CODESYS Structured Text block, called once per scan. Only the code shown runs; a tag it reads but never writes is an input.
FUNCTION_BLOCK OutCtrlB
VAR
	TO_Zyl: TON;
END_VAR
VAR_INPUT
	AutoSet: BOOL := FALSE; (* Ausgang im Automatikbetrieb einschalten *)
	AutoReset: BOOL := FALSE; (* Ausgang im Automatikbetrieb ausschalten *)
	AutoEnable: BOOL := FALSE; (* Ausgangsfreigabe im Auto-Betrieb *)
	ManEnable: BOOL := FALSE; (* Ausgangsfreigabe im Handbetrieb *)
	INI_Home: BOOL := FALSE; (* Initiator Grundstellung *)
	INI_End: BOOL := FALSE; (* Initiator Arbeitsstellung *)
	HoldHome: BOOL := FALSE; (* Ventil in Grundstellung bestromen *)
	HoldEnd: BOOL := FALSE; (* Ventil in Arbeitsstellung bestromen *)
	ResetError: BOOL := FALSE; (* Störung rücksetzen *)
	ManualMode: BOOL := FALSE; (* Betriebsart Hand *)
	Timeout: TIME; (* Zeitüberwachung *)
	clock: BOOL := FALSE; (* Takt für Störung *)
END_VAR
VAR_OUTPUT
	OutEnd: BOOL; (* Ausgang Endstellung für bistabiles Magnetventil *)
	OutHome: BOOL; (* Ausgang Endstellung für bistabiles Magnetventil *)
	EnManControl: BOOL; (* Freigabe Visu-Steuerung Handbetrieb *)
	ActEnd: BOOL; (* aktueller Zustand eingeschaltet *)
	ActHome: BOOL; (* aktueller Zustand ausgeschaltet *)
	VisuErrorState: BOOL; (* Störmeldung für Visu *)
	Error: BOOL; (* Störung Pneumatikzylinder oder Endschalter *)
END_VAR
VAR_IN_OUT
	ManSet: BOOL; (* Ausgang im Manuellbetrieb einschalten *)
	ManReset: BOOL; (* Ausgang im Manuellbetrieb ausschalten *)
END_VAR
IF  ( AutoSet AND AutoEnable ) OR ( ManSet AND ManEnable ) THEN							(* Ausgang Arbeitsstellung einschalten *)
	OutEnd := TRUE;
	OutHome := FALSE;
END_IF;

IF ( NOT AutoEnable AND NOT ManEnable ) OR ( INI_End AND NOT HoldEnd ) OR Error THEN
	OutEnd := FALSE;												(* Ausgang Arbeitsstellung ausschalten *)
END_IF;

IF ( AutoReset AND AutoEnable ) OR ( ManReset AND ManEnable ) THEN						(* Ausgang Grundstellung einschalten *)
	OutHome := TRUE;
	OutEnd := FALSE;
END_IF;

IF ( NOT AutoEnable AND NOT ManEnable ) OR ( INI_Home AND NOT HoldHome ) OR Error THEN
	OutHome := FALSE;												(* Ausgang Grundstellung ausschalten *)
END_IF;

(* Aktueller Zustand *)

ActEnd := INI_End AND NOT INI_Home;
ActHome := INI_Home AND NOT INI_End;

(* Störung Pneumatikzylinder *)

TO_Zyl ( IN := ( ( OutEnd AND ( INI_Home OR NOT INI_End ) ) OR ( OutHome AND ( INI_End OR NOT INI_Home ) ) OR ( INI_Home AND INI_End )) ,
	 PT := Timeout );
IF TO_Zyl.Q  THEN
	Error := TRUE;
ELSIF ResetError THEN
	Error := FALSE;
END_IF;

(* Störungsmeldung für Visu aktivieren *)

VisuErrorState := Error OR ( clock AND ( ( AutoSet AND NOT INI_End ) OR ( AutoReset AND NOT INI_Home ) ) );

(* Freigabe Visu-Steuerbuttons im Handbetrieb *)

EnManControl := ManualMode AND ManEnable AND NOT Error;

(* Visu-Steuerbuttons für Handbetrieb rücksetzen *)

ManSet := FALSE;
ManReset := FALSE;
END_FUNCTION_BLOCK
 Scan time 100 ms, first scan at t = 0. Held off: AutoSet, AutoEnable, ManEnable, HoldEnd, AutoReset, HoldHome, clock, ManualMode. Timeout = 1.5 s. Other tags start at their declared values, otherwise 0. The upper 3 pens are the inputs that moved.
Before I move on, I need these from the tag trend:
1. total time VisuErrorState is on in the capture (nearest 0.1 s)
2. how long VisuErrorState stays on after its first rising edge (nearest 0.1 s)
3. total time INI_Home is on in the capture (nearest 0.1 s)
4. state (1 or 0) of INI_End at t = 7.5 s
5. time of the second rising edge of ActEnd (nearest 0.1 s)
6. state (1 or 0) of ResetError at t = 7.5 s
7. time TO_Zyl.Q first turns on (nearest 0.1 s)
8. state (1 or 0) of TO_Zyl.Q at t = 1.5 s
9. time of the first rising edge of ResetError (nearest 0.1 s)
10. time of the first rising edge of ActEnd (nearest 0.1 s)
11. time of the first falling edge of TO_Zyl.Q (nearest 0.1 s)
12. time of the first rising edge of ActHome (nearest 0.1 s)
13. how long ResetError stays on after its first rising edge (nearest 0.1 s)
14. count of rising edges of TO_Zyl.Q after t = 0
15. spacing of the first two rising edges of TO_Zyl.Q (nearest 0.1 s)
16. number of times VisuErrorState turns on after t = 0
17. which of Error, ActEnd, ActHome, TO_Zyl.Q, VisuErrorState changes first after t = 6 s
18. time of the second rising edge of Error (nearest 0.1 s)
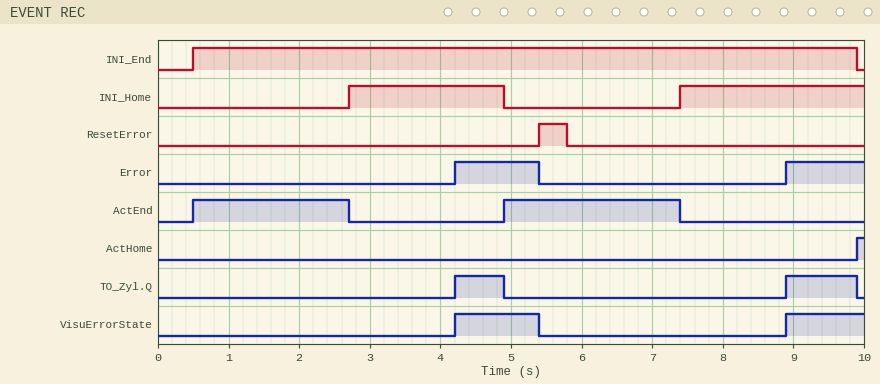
2.3 s
1.2 s
4.8 s
1
4.9 s
0
4.2 s
0
5.4 s
0.5 s
4.9 s
9.9 s
0.4 s
2
4.7 s
2
ActEnd
8.9 s
